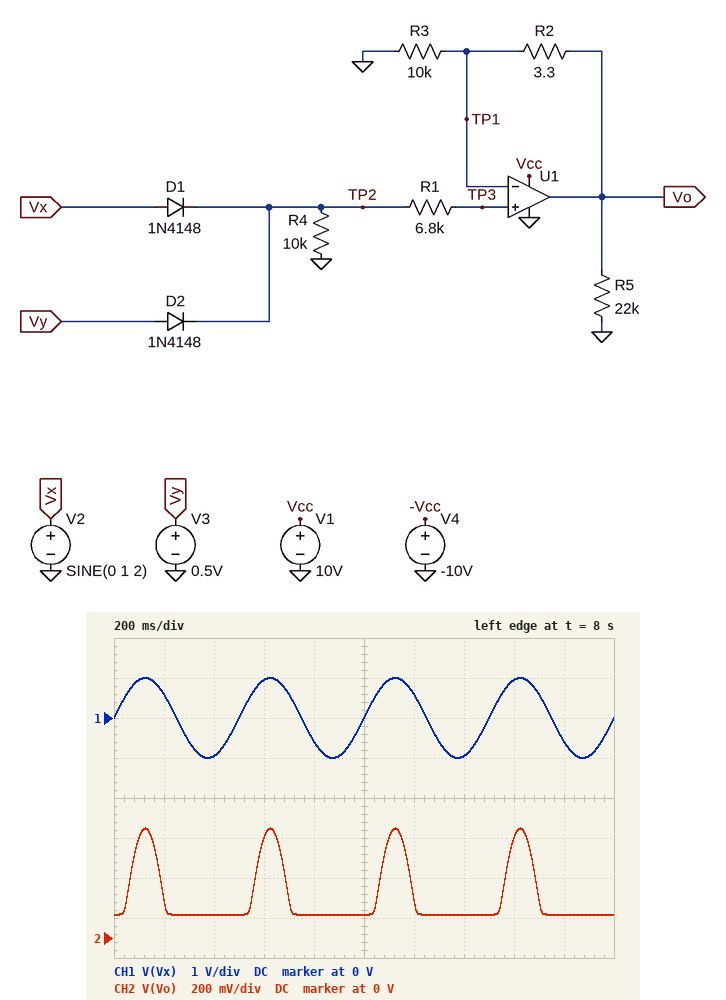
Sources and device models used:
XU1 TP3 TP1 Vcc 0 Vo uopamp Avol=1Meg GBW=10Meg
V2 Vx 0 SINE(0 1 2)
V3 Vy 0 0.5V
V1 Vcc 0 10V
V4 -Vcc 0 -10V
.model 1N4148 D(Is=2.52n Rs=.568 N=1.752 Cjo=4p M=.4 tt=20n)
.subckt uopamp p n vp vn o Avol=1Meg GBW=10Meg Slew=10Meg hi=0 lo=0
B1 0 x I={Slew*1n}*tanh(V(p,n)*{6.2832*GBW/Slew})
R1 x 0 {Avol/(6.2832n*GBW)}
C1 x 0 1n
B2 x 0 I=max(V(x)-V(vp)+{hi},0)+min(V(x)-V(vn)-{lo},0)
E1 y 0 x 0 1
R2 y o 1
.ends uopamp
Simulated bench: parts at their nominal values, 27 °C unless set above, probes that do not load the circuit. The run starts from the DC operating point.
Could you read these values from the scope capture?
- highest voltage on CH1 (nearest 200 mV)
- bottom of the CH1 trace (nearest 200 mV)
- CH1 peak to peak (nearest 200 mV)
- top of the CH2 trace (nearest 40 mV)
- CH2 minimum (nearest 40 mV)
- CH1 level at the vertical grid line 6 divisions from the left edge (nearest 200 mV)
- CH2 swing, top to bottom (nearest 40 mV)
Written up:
1.0 V
-1.0 V
2.0 V
560 mV
120 mV
600 mV
440 mV
